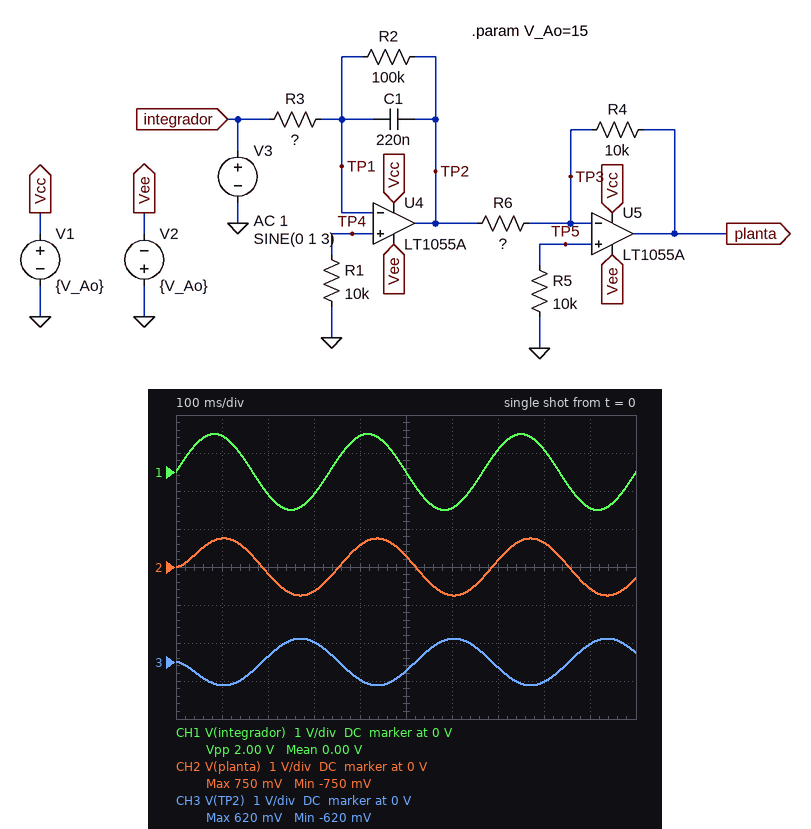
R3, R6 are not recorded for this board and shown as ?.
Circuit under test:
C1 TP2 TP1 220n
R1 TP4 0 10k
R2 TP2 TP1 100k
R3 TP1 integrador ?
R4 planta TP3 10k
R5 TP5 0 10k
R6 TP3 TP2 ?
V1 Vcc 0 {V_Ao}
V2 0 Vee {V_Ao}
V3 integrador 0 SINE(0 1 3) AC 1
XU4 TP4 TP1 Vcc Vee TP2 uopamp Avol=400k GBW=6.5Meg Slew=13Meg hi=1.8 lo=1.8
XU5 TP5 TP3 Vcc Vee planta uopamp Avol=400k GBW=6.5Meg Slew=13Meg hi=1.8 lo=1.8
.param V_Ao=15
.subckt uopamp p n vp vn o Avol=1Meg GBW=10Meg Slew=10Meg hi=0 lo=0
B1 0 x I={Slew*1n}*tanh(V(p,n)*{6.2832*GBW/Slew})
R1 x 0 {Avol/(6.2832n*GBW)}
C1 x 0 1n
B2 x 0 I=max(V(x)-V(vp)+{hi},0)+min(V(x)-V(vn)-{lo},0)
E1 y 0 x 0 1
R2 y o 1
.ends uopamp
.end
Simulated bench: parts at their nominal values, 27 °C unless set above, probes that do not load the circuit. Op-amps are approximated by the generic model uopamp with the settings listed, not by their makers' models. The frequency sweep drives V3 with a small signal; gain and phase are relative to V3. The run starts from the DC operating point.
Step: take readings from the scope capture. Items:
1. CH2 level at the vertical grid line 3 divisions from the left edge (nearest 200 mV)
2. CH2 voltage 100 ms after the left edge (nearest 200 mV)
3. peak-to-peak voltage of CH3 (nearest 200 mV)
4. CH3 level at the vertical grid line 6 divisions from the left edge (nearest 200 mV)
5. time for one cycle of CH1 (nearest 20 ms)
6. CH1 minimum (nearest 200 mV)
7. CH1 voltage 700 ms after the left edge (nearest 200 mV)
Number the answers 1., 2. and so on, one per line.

1. -600 mV
2. 800 mV
3. 1.2 V
4. 600 mV
5. 340 ms
6. -1.0 V
7. 600 mV
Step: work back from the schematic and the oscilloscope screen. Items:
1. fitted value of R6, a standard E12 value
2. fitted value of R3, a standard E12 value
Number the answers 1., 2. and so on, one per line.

1. 8.2 kΩ
2. 150 kΩ
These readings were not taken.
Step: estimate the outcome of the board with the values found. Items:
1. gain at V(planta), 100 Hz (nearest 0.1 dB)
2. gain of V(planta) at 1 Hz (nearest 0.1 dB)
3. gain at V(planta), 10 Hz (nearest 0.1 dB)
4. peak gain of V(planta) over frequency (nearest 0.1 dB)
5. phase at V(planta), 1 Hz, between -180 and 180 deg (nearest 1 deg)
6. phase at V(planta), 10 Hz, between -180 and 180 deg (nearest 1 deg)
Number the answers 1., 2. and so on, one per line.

1. -24.6 dB
2. -1.9 dB
3. -6.4 dB
4. -1.8 dB
5. -8 deg
6. -54 deg
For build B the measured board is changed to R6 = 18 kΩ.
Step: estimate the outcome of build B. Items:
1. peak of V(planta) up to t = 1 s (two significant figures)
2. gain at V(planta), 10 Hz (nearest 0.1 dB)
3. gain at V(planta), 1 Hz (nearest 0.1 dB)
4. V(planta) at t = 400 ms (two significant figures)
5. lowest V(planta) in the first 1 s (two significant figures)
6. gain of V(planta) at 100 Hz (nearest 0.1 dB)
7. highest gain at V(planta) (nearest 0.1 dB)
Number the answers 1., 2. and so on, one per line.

1. 340 mV
2. -13.3 dB
3. -8.7 dB
4. 260 mV
5. -340 mV
6. -31.5 dB
7. -8.6 dB
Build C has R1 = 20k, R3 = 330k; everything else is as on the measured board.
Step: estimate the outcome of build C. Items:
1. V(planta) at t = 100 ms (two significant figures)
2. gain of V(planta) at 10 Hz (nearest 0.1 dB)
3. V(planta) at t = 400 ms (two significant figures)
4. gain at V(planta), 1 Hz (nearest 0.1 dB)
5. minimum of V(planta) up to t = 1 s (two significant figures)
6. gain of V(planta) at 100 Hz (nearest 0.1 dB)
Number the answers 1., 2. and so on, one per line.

1. 340 mV
2. -13.3 dB
3. 260 mV
4. -8.7 dB
5. -340 mV
6. -31.5 dB
